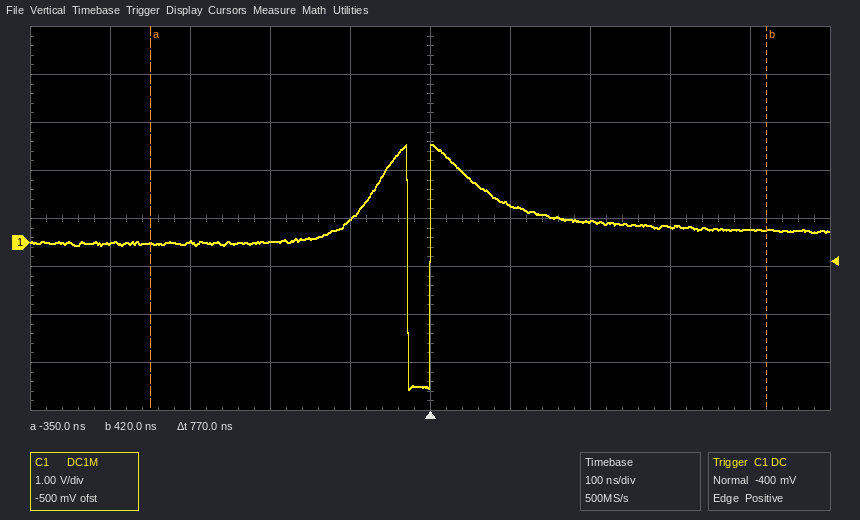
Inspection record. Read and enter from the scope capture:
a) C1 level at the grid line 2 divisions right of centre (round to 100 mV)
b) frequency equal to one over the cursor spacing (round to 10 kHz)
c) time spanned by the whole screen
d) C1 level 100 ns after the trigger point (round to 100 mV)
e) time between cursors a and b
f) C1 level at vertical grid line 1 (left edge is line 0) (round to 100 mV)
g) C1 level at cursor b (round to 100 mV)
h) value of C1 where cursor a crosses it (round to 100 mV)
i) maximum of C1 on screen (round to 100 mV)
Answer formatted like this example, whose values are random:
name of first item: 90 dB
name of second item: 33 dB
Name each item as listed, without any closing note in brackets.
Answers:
C1 level at the grid line 2 divisions right of centre: 400 mV
frequency equal to one over the cursor spacing: 1.30 MHz
time spanned by the whole screen: 1 µs
C1 level 100 ns after the trigger point: 800 mV
time between cursors a and b: 770 ns
C1 level at vertical grid line 1 (left edge is line 0): 0.0 V
C1 level at cursor b: 300 mV
value of C1 where cursor a crosses it: 0.0 V
maximum of C1 on screen: 2.0 V
